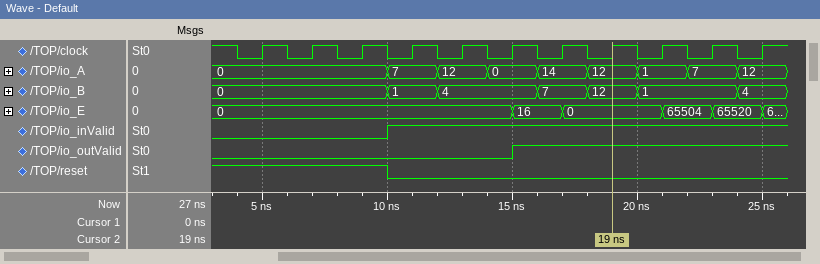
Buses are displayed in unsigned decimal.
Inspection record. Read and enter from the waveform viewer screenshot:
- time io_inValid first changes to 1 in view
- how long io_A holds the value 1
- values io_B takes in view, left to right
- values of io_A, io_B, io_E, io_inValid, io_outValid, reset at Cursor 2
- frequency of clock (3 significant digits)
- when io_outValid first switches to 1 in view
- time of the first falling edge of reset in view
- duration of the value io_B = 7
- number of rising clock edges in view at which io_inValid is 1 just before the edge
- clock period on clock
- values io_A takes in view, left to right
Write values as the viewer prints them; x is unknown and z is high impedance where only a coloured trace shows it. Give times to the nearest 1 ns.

10 ns
2 ns
0, 1, 4, 7, 12, 1, 4
io_A=12, io_B=12, io_E=0, io_inValid=1, io_outValid=1, reset=0
500 MHz
15 ns
10 ns
2 ns
8
2 ns
0, 7, 12, 0, 14, 12, 1, 7, 12
